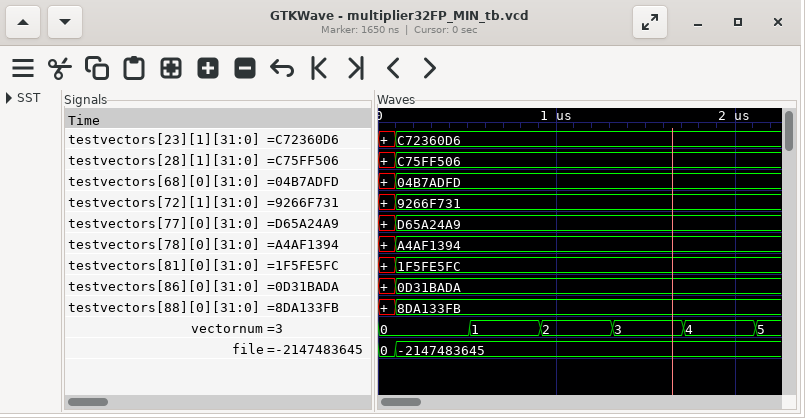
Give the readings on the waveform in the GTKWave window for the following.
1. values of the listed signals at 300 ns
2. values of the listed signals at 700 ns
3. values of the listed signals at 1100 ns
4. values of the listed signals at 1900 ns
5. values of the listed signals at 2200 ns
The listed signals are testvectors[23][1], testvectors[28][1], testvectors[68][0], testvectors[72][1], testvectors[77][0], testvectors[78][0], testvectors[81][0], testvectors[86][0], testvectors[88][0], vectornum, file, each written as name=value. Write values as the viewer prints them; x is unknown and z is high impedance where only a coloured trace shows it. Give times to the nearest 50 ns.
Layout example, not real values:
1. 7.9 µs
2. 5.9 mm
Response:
1. testvectors[23][1]=C72360D6, testvectors[28][1]=C75FF506, testvectors[68][0]=04B7ADFD, testvectors[72][1]=9266F731, testvectors[77][0]=D65A24A9, testvectors[78][0]=A4AF1394, testvectors[81][0]=1F5FE5FC, testvectors[86][0]=0D31BADA, testvectors[88][0]=8DA133FB, vectornum=0, file=-2147483645
2. testvectors[23][1]=C72360D6, testvectors[28][1]=C75FF506, testvectors[68][0]=04B7ADFD, testvectors[72][1]=9266F731, testvectors[77][0]=D65A24A9, testvectors[78][0]=A4AF1394, testvectors[81][0]=1F5FE5FC, testvectors[86][0]=0D31BADA, testvectors[88][0]=8DA133FB, vectornum=1, file=-2147483645
3. testvectors[23][1]=C72360D6, testvectors[28][1]=C75FF506, testvectors[68][0]=04B7ADFD, testvectors[72][1]=9266F731, testvectors[77][0]=D65A24A9, testvectors[78][0]=A4AF1394, testvectors[81][0]=1F5FE5FC, testvectors[86][0]=0D31BADA, testvectors[88][0]=8DA133FB, vectornum=2, file=-2147483645
4. testvectors[23][1]=C72360D6, testvectors[28][1]=C75FF506, testvectors[68][0]=04B7ADFD, testvectors[72][1]=9266F731, testvectors[77][0]=D65A24A9, testvectors[78][0]=A4AF1394, testvectors[81][0]=1F5FE5FC, testvectors[86][0]=0D31BADA, testvectors[88][0]=8DA133FB, vectornum=4, file=-2147483645
5. testvectors[23][1]=C72360D6, testvectors[28][1]=C75FF506, testvectors[68][0]=04B7ADFD, testvectors[72][1]=9266F731, testvectors[77][0]=D65A24A9, testvectors[78][0]=A4AF1394, testvectors[81][0]=1F5FE5FC, testvectors[86][0]=0D31BADA, testvectors[88][0]=8DA133FB, vectornum=5, file=-2147483645
